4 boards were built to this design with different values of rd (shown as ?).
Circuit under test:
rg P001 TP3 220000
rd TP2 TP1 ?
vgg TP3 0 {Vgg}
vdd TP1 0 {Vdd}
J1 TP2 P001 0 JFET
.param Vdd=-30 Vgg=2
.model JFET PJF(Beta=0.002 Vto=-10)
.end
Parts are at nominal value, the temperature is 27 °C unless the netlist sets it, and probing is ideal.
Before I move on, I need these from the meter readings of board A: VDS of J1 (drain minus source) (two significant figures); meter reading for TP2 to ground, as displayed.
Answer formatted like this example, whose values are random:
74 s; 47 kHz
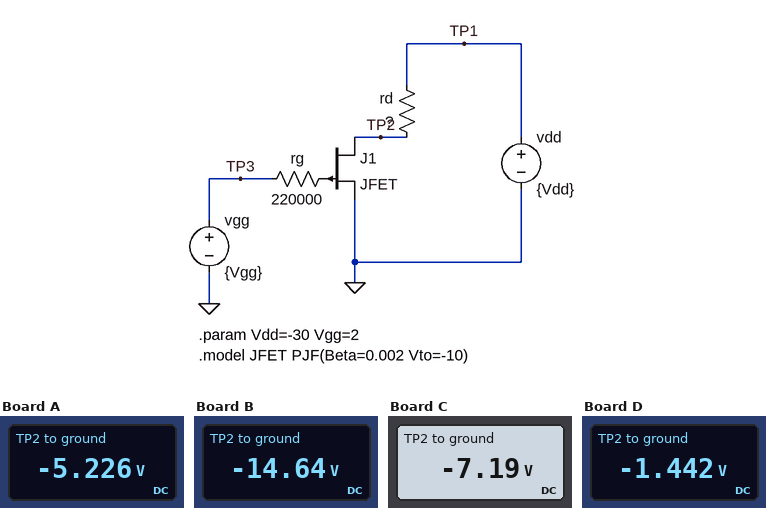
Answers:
-5.2 V; -5.226 V
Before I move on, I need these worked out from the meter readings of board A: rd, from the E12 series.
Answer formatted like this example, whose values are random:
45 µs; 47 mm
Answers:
220 Ω
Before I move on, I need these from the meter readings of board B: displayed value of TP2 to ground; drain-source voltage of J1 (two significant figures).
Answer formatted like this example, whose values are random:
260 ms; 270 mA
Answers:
-14.64 V; -15 V
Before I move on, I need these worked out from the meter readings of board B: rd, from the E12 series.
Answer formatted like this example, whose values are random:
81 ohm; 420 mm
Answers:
120 Ω
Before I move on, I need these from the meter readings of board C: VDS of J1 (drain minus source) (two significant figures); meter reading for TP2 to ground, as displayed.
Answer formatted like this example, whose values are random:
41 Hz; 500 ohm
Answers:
-7.2 V; -7.19 V
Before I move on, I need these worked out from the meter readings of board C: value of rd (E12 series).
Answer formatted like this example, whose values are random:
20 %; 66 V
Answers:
180 Ω
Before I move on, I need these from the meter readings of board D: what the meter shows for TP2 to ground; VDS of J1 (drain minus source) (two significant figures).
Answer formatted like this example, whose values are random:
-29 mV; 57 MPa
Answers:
-1.442 V; -1.4 V
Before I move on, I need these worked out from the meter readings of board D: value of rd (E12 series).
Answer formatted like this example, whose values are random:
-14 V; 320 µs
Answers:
680 Ω
